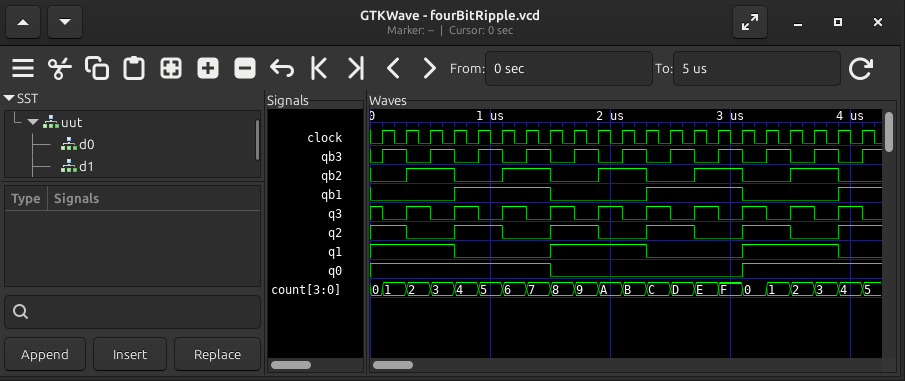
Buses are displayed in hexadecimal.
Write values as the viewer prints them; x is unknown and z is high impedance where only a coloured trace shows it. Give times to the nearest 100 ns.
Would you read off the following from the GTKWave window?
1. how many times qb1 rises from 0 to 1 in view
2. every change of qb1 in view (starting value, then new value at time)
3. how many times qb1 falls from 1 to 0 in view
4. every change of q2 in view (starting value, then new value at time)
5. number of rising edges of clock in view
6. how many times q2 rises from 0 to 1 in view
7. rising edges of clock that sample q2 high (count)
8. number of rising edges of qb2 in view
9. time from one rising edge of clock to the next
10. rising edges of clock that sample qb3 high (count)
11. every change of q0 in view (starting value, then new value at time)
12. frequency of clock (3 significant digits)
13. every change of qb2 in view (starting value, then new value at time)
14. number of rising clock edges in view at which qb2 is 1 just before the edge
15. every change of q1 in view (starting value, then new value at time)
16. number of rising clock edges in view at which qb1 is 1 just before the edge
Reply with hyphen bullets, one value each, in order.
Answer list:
- 3
- 0, 1 at 700 ns, 0 at 1500 ns, 1 at 2300 ns, 0 at 3100 ns, 1 at 3900 ns
- 2
- 1, 0 at 300 ns, 1 at 700 ns, 0 at 1100 ns, 1 at 1500 ns, 0 at 1900 ns, 1 at 2300 ns, 0 at 2700 ns, 1 at 3100 ns, 0 at 3500 ns, 1 at 3900 ns
- 21
- 5
- 11
- 5
- 200 ns
- 10
- 1, 0 at 1500 ns, 1 at 3100 ns
- 5.00 MHz
- 0, 1 at 300 ns, 0 at 700 ns, 1 at 1100 ns, 0 at 1500 ns, 1 at 1900 ns, 0 at 2300 ns, 1 at 2700 ns, 0 at 3100 ns, 1 at 3500 ns, 0 at 3900 ns
- 10
- 1, 0 at 700 ns, 1 at 1500 ns, 0 at 2300 ns, 1 at 3100 ns, 0 at 3900 ns
- 9
